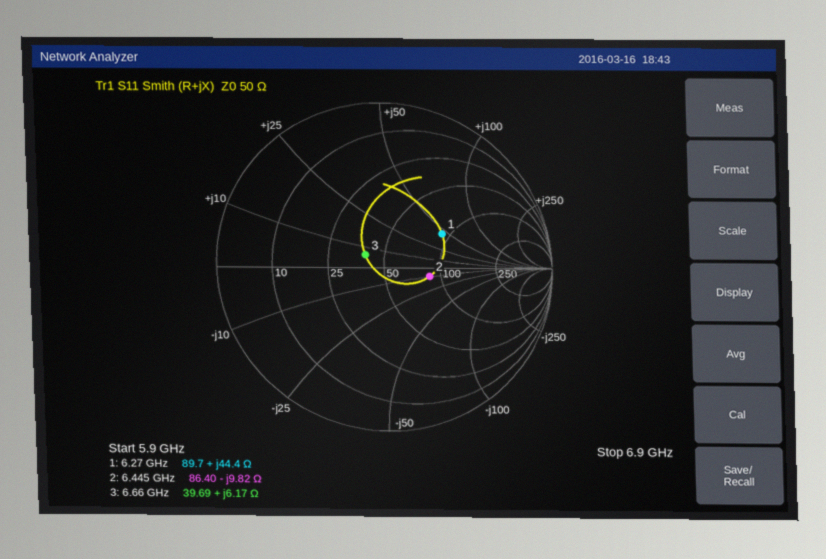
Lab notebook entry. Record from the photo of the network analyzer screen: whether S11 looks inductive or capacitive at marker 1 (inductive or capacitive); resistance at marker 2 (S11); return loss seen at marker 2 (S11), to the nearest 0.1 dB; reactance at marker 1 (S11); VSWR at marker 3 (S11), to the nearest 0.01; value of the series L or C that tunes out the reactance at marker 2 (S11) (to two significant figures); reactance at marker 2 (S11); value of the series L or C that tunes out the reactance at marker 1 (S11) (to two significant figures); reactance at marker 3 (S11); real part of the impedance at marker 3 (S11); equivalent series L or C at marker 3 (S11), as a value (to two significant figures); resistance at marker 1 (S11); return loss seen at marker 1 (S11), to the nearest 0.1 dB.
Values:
inductive
86.40 Ω
11.2 dB
+44.4 Ω
1.31
240 pH
-9.82 Ω
570 fF
+6.17 Ω
39.69 Ω
150 pH
89.7 Ω
7.8 dB
